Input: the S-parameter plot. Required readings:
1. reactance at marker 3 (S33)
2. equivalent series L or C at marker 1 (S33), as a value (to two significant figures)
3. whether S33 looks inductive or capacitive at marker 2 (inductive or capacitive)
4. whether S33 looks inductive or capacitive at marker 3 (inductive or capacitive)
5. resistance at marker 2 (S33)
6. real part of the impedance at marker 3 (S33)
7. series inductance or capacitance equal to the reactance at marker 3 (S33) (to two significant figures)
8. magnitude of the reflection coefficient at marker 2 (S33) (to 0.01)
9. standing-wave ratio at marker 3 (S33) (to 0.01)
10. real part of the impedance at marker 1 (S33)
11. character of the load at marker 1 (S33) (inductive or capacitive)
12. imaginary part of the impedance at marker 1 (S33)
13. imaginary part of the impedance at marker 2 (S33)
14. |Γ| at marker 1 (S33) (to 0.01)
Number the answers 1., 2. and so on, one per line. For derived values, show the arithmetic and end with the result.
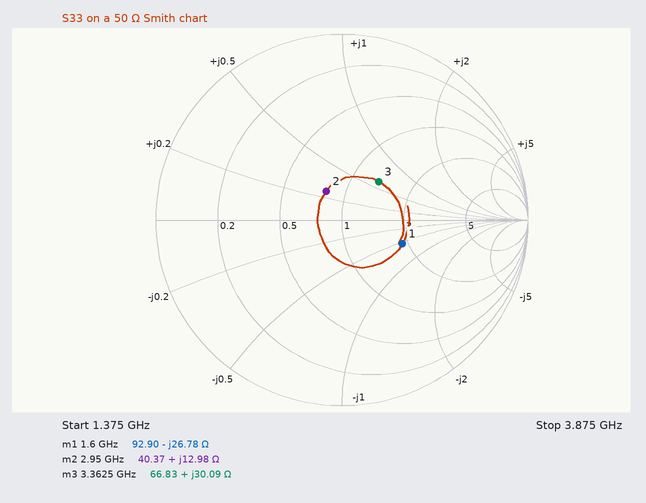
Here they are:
1. +30.09 Ω
2. C = 1/(2π × 1.6 GHz × 26.78 Ω) ≈ 3.7 pF
3. inductive
4. inductive
5. 40.37 Ω
6. 66.83 Ω
7. L = 30.09 Ω/(2π × 3.3625 GHz) ≈ 1.4 nH
8. 0.18
9. 1.80
10. 92.90 Ω
11. capacitive
12. -26.78 Ω
13. +12.98 Ω
14. 0.35
